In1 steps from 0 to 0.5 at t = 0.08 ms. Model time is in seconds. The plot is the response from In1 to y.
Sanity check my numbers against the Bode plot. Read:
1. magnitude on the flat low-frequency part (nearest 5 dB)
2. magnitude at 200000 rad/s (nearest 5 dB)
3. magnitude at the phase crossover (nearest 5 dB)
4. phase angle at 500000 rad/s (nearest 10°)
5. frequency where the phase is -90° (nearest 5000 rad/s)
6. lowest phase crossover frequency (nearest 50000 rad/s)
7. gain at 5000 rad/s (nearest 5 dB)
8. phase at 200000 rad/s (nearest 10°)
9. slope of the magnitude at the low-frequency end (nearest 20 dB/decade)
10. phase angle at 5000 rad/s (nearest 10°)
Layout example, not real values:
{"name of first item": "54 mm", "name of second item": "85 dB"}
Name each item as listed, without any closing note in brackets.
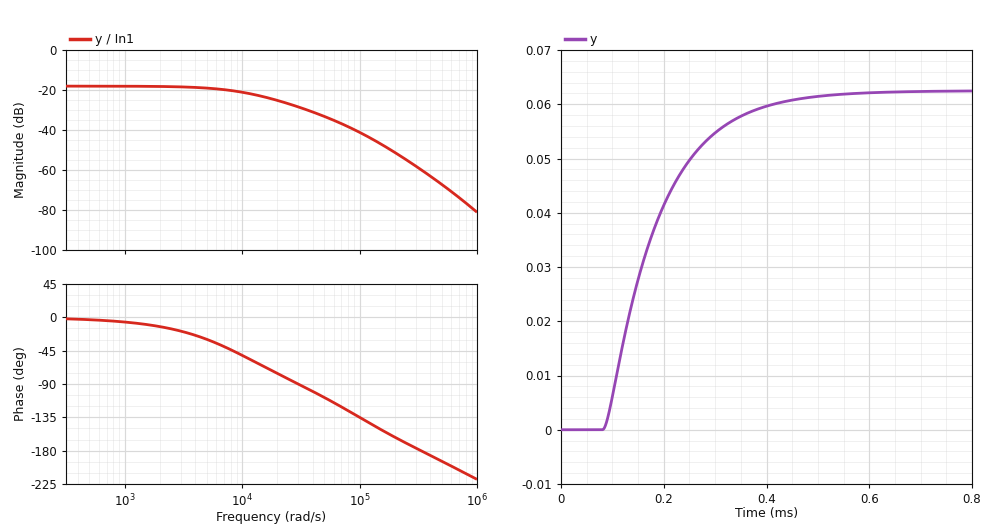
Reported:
{"magnitude on the flat low-frequency part": "-20 dB", "magnitude at 200000 rad/s": "-50 dB", "magnitude at the phase crossover": "-60 dB", "phase angle at 500000 rad/s": "-190°", "frequency where the phase is -90°": "30000 rad/s", "lowest phase crossover frequency": "350000 rad/s", "gain at 5000 rad/s": "-20 dB", "phase at 200000 rad/s": "-160°", "slope of the magnitude at the low-frequency end": "0 dB/decade", "phase angle at 5000 rad/s": "-30°"}
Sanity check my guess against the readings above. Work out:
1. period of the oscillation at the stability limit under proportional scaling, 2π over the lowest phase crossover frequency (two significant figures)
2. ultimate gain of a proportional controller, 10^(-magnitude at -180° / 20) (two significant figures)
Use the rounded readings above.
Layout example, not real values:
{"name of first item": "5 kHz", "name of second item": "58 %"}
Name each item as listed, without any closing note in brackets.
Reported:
{"period of the oscillation at the stability limit under proportional scaling, 2π over the lowest phase crossover frequency": "0.000018 s", "ultimate gain of a proportional controller, 10^(-magnitude at -180° / 20)": "1000"}
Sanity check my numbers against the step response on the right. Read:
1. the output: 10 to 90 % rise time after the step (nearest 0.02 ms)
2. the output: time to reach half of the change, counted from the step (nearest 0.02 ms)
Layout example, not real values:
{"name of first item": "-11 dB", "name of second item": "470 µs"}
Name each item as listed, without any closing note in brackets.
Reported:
{"the output: 10 to 90 % rise time after the step": "0.22 ms", "the output: time to reach half of the change, counted from the step": "0.08 ms"}
